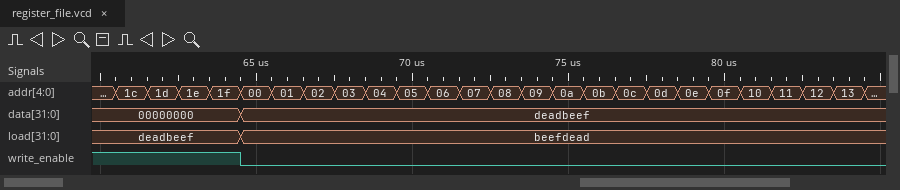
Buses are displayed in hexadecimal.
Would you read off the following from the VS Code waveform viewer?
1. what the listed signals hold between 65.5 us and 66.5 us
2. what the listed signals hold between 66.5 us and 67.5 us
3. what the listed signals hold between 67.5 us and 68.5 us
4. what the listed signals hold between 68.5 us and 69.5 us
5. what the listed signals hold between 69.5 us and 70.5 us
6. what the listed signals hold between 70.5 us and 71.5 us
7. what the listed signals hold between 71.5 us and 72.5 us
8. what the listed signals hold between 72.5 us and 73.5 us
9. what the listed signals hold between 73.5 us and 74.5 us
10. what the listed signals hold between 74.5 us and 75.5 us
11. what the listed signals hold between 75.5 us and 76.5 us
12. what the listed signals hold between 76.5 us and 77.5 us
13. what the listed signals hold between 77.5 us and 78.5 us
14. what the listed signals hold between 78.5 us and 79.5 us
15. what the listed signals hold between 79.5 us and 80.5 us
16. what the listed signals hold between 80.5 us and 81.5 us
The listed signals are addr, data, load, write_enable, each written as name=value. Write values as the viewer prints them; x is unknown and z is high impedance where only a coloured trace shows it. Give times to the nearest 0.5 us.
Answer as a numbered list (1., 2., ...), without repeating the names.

1. addr=01, data=deadbeef, load=beefdead, write_enable=0
2. addr=02, data=deadbeef, load=beefdead, write_enable=0
3. addr=03, data=deadbeef, load=beefdead, write_enable=0
4. addr=04, data=deadbeef, load=beefdead, write_enable=0
5. addr=05, data=deadbeef, load=beefdead, write_enable=0
6. addr=06, data=deadbeef, load=beefdead, write_enable=0
7. addr=07, data=deadbeef, load=beefdead, write_enable=0
8. addr=08, data=deadbeef, load=beefdead, write_enable=0
9. addr=09, data=deadbeef, load=beefdead, write_enable=0
10. addr=0a, data=deadbeef, load=beefdead, write_enable=0
11. addr=0b, data=deadbeef, load=beefdead, write_enable=0
12. addr=0c, data=deadbeef, load=beefdead, write_enable=0
13. addr=0d, data=deadbeef, load=beefdead, write_enable=0
14. addr=0e, data=deadbeef, load=beefdead, write_enable=0
15. addr=0f, data=deadbeef, load=beefdead, write_enable=0
16. addr=10, data=deadbeef, load=beefdead, write_enable=0
